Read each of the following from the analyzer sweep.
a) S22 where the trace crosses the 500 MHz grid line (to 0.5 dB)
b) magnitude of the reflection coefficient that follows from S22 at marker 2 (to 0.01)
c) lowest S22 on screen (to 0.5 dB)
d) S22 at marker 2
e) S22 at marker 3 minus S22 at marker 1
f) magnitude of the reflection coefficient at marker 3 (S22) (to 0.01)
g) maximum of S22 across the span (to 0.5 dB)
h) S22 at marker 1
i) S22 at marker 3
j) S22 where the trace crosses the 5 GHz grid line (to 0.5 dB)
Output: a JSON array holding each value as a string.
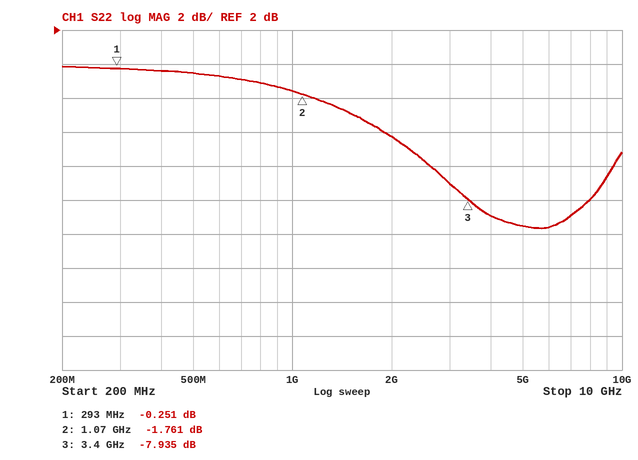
["-0.5 dB", "0.82", "-9.5 dB", "-1.761 dB", "-7.684 dB", "0.40", "0.0 dB", "-0.251 dB", "-7.935 dB", "-9.5 dB"]
